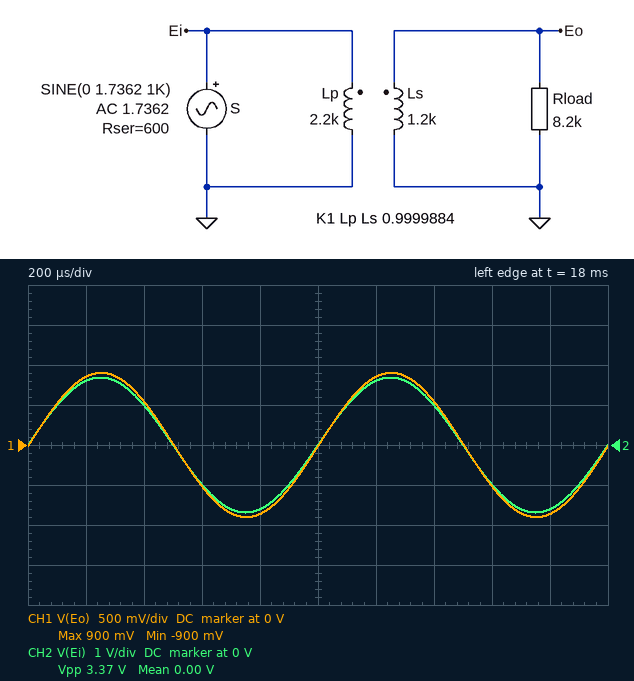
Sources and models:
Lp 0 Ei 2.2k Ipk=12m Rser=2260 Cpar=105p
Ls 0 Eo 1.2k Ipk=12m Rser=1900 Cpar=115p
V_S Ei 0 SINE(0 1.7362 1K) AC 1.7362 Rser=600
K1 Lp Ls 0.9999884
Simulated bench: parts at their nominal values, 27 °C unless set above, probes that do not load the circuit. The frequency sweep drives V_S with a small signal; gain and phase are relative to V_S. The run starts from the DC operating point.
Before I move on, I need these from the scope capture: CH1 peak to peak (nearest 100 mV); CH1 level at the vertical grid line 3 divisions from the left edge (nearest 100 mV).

1.8 V
-500 mV
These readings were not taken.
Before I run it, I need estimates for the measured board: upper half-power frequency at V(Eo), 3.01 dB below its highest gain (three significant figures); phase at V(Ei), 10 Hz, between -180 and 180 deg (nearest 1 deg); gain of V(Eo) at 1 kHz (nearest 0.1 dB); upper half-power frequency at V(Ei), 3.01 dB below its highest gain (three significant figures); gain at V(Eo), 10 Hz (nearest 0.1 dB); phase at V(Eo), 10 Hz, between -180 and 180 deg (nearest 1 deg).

80.5 kHz
0 deg
-5.7 dB
2.55 MHz
-5.7 dB
1 deg
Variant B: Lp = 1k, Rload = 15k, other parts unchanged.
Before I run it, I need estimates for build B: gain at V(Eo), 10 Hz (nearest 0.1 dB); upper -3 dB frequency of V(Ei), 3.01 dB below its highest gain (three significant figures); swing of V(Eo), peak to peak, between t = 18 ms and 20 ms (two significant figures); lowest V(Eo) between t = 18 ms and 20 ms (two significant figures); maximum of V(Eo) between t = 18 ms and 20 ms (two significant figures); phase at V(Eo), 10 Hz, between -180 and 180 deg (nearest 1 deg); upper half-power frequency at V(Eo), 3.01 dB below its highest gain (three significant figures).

-1.9 dB
2.56 MHz
2.8 V
-1.4 V
1.4 V
2 deg
116 kHz
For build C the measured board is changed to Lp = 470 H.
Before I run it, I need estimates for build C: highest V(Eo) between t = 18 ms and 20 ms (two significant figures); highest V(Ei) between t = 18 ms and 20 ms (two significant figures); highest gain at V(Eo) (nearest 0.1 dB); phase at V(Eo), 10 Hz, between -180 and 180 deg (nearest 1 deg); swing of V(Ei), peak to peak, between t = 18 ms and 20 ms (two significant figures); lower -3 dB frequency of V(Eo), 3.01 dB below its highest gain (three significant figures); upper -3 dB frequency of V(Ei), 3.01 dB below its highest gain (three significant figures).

1.3 V
1.6 V
-2.5 dB
3 deg
3.2 V
562 mHz
2.58 MHz
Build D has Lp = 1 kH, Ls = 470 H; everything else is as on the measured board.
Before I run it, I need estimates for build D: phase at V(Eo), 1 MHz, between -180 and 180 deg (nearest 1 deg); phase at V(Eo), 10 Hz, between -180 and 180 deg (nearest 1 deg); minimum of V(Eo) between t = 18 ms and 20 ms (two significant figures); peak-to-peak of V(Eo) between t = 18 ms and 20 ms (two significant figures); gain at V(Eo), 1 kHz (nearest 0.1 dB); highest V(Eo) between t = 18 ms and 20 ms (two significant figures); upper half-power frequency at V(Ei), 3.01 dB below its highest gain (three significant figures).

171 deg
2 deg
-850 mV
1.7 V
-6.2 dB
850 mV
2.58 MHz
